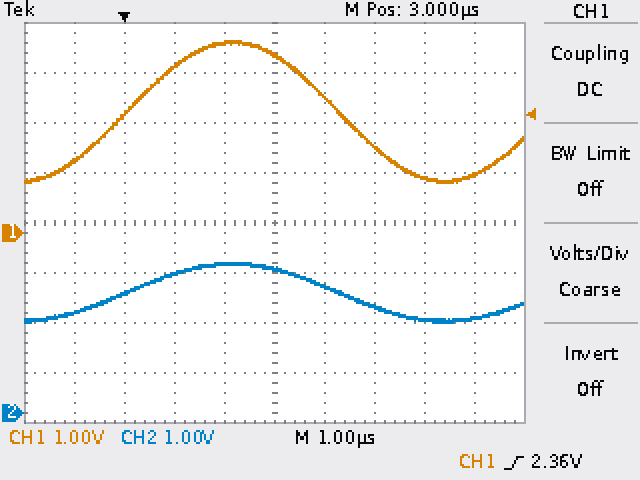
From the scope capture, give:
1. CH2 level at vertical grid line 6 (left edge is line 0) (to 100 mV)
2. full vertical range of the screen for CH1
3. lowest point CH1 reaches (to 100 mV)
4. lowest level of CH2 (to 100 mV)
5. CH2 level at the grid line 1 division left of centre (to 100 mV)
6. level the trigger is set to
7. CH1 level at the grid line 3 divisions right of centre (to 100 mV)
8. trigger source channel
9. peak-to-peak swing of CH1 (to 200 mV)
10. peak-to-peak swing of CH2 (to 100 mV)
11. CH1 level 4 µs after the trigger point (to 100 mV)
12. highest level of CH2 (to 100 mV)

2.5 V
8 V
1.0 V
1.8 V
3.0 V
2.36 V
1.1 V
CH1
2.8 V
1.2 V
2.7 V
3.0 V
